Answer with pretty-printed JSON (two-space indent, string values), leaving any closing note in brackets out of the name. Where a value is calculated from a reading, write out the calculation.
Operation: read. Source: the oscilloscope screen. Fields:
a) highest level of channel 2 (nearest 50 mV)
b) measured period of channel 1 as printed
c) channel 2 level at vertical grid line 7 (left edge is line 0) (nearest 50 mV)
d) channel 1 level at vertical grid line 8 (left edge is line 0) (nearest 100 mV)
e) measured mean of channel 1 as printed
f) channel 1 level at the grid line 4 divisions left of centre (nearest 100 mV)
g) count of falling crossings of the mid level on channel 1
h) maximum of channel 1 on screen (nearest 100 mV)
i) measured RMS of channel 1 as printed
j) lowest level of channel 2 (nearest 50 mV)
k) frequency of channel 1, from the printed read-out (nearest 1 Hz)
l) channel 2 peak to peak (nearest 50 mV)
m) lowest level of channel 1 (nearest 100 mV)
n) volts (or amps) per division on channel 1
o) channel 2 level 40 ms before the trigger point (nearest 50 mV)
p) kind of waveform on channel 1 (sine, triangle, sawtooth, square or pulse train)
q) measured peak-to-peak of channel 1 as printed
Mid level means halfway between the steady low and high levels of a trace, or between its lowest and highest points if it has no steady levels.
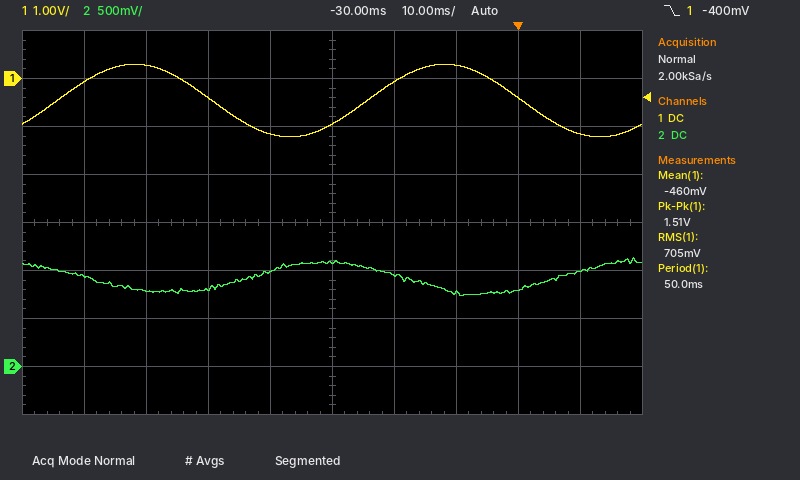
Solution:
{
  "highest level of channel 2": "1.15 V",
  "measured period of channel 1 as printed": "50.0 ms",
  "channel 2 level at vertical grid line 7 (left edge is line 0)": "750 mV",
  "channel 1 level at vertical grid line 8 (left edge is line 0)": "-400 mV",
  "measured mean of channel 1 as printed": "-460 mV",
  "channel 1 level at the grid line 4 divisions left of centre": "-100 mV",
  "count of falling crossings of the mid level on channel 1": "2",
  "maximum of channel 1 on screen": "300 mV",
  "measured RMS of channel 1 as printed": "705 mV",
  "lowest level of channel 2": "750 mV",
  "frequency of channel 1, from the printed read-out": "1 / 50.0 ms ≈ 20 Hz",
  "channel 2 peak to peak": "1.15 V − (750 mV) = 400 mV",
  "lowest level of channel 1": "-1.2 V",
  "volts (or amps) per division on channel 1": "1 V",
  "channel 2 level 40 ms before the trigger point": "1.00 V",
  "kind of waveform on channel 1": "sine",
  "measured peak-to-peak of channel 1 as printed": "1.51 V"
}
